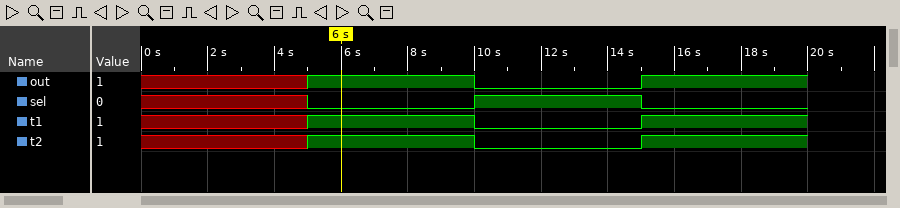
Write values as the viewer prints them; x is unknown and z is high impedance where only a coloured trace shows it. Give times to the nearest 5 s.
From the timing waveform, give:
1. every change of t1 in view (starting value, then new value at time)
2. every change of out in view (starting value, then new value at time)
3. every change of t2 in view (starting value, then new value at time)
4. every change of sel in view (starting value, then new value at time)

x, 1 at 5 s, 0 at 10 s, 1 at 15 s
x, 1 at 5 s, 0 at 10 s, 1 at 15 s
x, 1 at 5 s, 0 at 10 s, 1 at 15 s
x, 0 at 5 s, 1 at 10 s, 0 at 15 s
